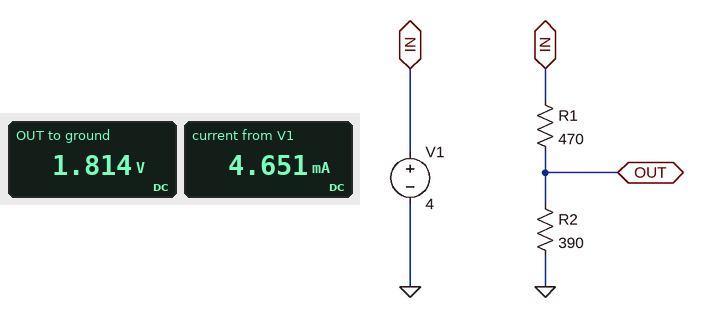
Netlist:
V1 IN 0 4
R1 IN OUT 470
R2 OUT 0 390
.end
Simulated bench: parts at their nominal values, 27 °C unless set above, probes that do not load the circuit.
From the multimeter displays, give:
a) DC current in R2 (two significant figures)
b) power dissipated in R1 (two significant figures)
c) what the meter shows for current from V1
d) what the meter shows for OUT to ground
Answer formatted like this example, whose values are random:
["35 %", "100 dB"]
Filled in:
["4.7 mA", "10 mW", "4.651 mA", "1.814 V"]
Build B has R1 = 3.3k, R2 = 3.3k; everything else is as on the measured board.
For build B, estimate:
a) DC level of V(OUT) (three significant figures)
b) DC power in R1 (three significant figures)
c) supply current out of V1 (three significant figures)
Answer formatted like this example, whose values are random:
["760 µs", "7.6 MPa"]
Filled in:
["2.00 V", "1.21 mW", "606 µA"]
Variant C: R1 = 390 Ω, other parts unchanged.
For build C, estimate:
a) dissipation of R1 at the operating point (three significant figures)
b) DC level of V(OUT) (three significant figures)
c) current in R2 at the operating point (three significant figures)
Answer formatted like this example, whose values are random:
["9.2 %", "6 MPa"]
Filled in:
["10.3 mW", "2.00 V", "5.13 mA"]
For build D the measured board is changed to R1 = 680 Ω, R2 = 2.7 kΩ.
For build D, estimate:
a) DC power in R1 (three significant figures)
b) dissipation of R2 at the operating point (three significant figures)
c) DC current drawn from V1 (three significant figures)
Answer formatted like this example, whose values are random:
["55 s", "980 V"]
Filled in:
["952 µW", "3.78 mW", "1.18 mA"]
